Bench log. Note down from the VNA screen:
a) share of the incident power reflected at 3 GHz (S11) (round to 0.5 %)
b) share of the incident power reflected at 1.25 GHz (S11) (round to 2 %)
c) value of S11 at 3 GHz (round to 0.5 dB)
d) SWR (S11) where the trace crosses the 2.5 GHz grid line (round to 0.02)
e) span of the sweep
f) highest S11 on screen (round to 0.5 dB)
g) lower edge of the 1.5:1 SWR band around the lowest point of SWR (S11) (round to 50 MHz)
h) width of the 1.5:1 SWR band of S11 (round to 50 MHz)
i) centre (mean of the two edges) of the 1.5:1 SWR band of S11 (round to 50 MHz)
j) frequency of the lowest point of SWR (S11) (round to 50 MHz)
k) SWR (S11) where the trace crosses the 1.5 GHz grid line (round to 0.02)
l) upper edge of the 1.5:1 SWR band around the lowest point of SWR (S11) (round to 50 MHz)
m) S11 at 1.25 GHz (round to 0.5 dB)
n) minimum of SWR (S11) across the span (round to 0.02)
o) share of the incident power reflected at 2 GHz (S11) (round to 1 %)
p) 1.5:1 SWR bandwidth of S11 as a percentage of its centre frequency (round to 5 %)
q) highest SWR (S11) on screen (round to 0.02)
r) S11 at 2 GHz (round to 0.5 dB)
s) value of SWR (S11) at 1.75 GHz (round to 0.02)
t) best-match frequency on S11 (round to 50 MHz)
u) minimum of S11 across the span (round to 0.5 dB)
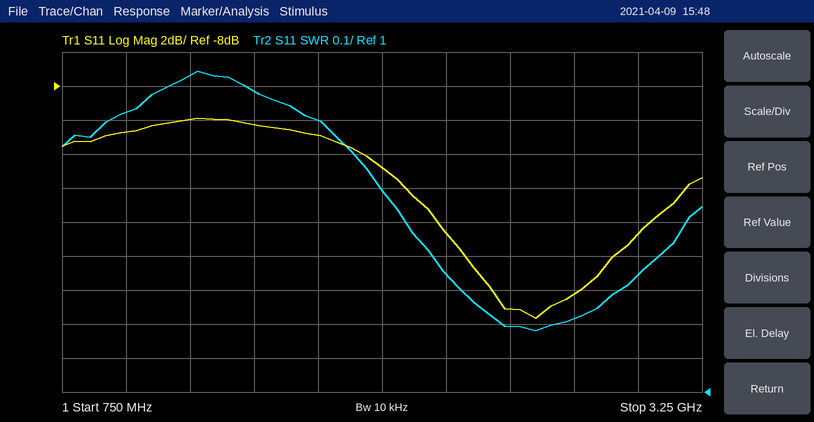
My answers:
2.0 %
10 %
-16.5 dB
1.20
2.5 GHz
-10.0 dB
2.10 GHz
1.10 GHz
2.65 GHz
2.60 GHz
1.88
3.20 GHz
-10.0 dB
1.18
5 %
40 %
1.94
-13.0 dB
1.80
2.60 GHz
-21.5 dB
